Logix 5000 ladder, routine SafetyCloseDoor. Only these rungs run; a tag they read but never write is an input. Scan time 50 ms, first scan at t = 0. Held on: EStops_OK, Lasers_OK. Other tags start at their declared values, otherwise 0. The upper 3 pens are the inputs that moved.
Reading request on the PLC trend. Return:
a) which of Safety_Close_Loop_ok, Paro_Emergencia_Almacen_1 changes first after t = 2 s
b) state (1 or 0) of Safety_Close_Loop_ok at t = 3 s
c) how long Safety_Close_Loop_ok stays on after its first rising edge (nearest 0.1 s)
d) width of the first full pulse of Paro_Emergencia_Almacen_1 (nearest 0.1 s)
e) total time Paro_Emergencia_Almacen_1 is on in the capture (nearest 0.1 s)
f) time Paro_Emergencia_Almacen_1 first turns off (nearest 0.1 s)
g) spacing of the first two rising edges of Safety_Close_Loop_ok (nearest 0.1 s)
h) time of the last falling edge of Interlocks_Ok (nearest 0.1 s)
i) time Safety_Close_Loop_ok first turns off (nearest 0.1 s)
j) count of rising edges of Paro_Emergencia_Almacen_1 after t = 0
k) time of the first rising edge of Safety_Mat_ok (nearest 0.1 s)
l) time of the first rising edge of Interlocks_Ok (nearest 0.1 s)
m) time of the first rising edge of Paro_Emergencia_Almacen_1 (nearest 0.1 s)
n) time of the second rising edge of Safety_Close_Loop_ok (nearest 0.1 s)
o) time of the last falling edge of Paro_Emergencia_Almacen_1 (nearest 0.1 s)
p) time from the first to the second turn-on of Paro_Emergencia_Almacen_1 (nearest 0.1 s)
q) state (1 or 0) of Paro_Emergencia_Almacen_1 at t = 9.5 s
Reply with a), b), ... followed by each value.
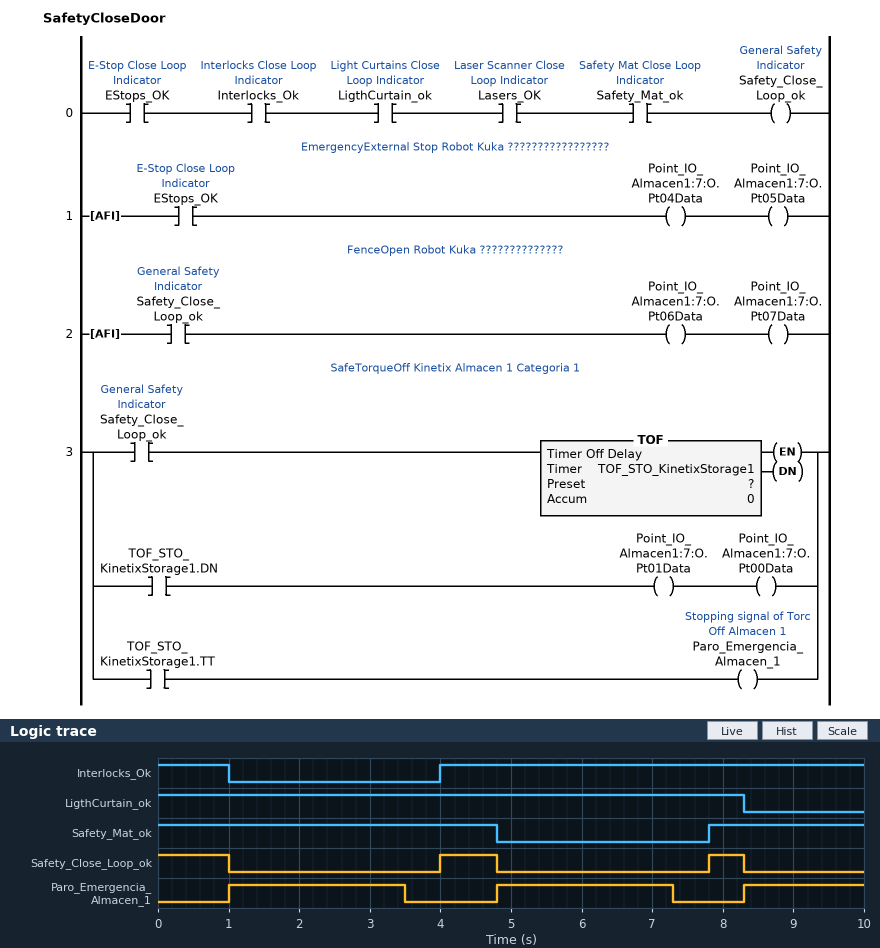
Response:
a) Paro_Emergencia_Almacen_1
b) 0
c) 0.8 s
d) 2.5 s
e) 6.7 s
f) 3.5 s
g) 3.8 s
h) 1.0 s
i) 1.0 s
j) 3
k) 7.8 s
l) 4.0 s
m) 1.0 s
n) 7.8 s
o) 7.3 s
p) 3.8 s
q) 1
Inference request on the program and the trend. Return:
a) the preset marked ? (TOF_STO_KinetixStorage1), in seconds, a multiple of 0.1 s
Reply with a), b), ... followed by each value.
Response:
a) 2.5 s
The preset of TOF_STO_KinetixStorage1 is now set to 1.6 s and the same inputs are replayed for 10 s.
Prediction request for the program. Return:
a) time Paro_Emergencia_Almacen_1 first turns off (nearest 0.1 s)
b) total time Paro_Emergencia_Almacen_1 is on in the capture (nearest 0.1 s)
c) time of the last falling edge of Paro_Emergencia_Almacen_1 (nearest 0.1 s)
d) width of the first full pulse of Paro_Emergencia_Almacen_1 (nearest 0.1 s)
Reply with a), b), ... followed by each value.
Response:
a) 2.6 s
b) 4.8 s
c) 9.9 s
d) 1.6 s
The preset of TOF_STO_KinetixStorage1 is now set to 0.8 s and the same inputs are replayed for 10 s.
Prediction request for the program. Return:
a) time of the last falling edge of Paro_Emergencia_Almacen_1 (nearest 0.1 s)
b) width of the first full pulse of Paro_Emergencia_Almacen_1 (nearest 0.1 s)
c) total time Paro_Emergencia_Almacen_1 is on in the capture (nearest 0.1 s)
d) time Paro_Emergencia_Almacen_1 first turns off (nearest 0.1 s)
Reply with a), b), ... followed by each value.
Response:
a) 9.1 s
b) 0.8 s
c) 2.4 s
d) 1.8 s
